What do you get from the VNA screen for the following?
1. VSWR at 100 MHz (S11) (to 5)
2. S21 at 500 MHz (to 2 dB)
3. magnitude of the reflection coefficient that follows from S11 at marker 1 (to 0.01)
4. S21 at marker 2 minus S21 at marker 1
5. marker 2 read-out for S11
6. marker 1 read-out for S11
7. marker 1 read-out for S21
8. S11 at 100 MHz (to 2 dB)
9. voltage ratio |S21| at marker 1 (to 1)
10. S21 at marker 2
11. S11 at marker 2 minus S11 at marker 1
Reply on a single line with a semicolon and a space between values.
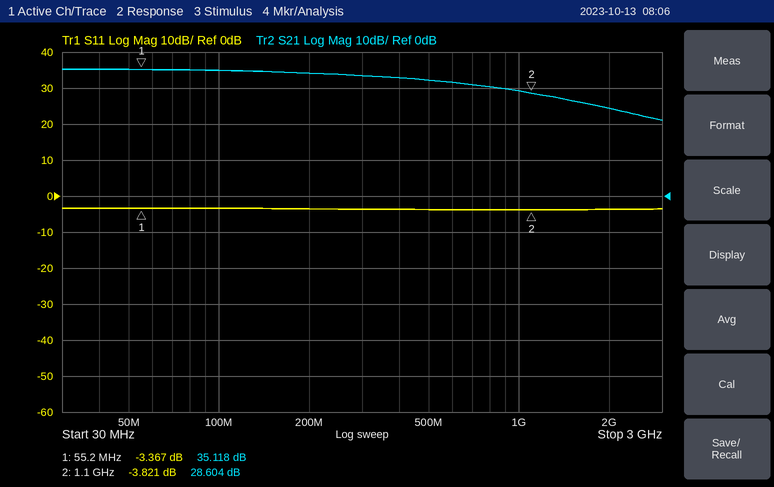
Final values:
5; 32 dB; 0.68; -6.514 dB; -3.821 dB; -3.367 dB; 35.118 dB; -4 dB; 57; 28.604 dB; -0.454 dB
